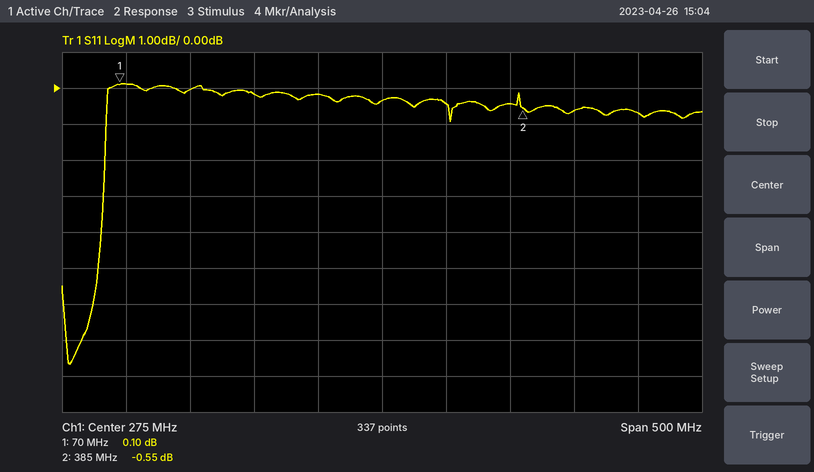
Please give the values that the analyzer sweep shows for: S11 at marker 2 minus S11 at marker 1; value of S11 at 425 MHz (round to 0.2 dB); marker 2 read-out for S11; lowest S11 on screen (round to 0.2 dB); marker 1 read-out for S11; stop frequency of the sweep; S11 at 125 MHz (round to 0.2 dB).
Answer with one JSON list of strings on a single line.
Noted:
["-0.65 dB", "-0.6 dB", "-0.55 dB", "-7.6 dB", "0.10 dB", "525 MHz", "0.0 dB"]
